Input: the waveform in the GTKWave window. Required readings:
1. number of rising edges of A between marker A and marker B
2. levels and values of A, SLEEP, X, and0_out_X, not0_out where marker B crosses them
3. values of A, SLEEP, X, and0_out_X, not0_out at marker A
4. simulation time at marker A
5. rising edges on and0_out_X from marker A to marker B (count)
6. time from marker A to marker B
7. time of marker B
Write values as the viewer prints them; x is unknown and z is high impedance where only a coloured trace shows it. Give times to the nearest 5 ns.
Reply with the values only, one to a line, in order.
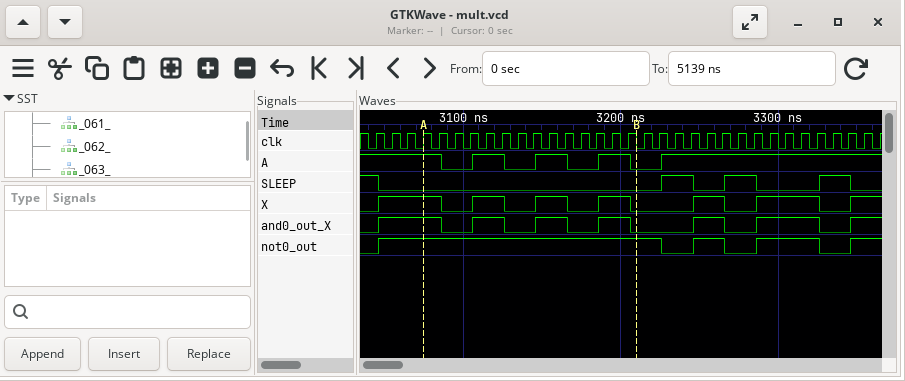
3
A=0, SLEEP=0, X=0, and0_out_X=0, not0_out=1
A=1, SLEEP=0, X=1, and0_out_X=1, not0_out=1
3075 ns
3
135 ns
3210 ns
